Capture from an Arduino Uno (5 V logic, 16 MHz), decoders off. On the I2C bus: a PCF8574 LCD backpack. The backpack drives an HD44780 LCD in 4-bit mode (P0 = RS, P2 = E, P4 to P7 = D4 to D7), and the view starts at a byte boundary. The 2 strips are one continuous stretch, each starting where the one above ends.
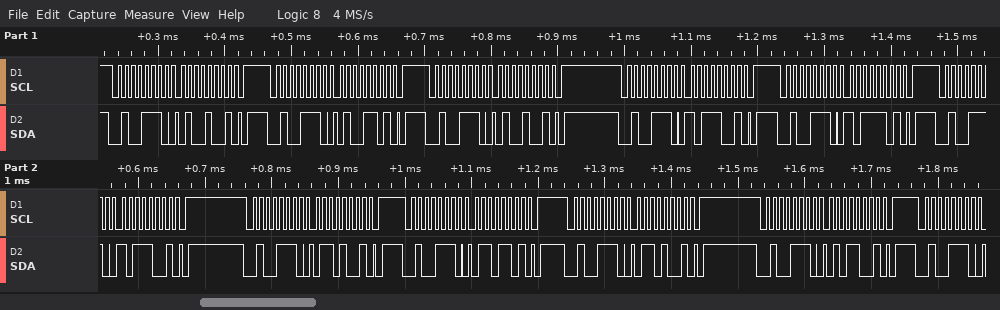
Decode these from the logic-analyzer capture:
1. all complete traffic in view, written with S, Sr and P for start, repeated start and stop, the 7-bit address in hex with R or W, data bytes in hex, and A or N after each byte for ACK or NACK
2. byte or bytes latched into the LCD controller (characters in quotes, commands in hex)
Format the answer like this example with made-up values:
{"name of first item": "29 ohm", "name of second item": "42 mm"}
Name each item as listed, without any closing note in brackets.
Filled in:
{"all complete traffic in view, written with S, Sr and P for start, repeated start and stop, the 7-bit address in hex with R or W, data bytes in hex, and A or N after each byte for ACK or NACK": "S 27W A 49 A P S 27W A 4D A P S 27W A 49 A P S 27W A B9 A P S 27W A BD A P S 27W A B9 A P S 27W A 69 A P S 27W A 6D A P S 27W A 69 A P S 27W A 59 A P S 27W A", "byte or bytes latched into the LCD controller": "'K'"}
